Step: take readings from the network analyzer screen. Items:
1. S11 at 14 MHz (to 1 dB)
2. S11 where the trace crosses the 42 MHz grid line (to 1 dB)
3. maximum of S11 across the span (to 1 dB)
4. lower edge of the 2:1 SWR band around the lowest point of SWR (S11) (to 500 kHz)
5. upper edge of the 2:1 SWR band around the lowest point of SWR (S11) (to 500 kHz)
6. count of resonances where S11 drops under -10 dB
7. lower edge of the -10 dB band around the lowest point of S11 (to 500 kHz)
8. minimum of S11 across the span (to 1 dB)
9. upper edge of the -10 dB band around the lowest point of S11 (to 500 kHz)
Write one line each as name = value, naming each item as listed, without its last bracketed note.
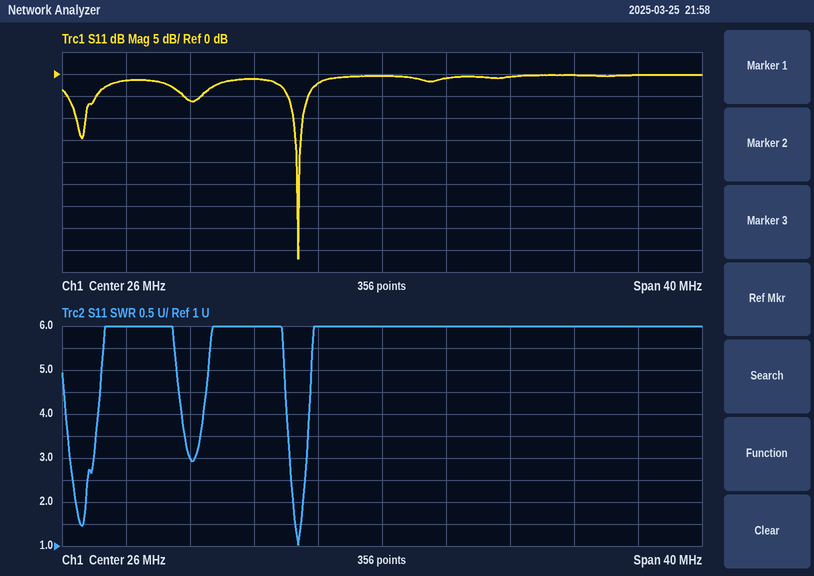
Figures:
S11 at 14 MHz = -6 dB
S11 where the trace crosses the 42 MHz grid line = 0 dB
maximum of S11 across the span = 0 dB
lower edge of the 2:1 SWR band around the lowest point of SWR (S11) = 20.5 MHz
upper edge of the 2:1 SWR band around the lowest point of SWR (S11) = 21.0 MHz
count of resonances where S11 drops under -10 dB = 2
lower edge of the -10 dB band around the lowest point of S11 = 20.5 MHz
minimum of S11 across the span = -42 dB
upper edge of the -10 dB band around the lowest point of S11 = 21.0 MHz
